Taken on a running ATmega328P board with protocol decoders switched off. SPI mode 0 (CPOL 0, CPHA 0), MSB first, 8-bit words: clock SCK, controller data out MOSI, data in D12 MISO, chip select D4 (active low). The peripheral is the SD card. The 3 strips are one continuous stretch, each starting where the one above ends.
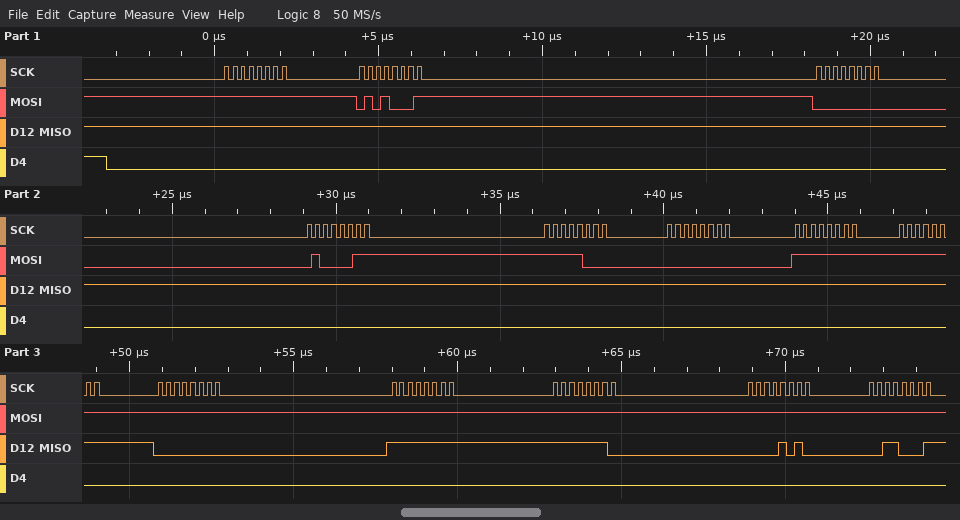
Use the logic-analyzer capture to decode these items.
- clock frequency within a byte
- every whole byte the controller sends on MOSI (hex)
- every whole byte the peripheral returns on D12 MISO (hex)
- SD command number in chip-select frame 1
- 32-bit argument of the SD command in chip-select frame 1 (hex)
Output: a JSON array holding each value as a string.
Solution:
["4 MHz", "FF 51 00 43 F8 00 FF FF FF FF FF FF FF", "FF FF FF FF FF FF FF FF 00 FF FE 0A 31", "CMD17", "0x0043F800"]
